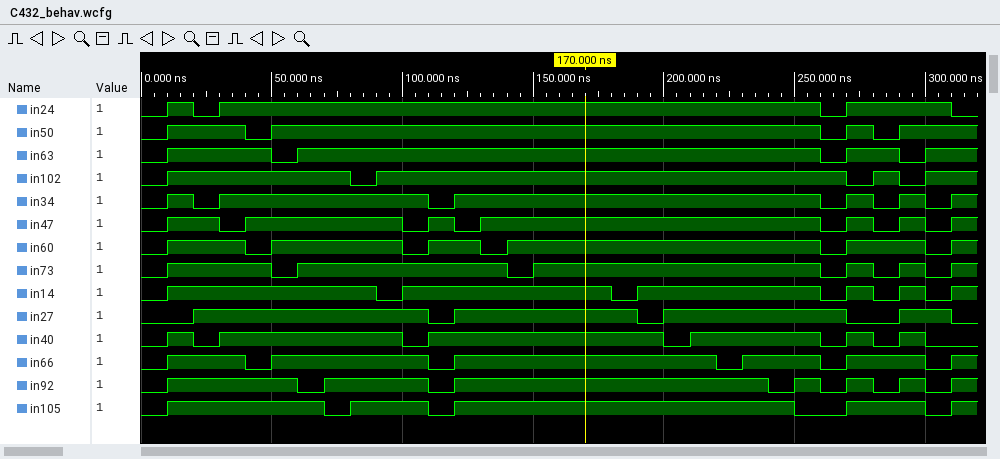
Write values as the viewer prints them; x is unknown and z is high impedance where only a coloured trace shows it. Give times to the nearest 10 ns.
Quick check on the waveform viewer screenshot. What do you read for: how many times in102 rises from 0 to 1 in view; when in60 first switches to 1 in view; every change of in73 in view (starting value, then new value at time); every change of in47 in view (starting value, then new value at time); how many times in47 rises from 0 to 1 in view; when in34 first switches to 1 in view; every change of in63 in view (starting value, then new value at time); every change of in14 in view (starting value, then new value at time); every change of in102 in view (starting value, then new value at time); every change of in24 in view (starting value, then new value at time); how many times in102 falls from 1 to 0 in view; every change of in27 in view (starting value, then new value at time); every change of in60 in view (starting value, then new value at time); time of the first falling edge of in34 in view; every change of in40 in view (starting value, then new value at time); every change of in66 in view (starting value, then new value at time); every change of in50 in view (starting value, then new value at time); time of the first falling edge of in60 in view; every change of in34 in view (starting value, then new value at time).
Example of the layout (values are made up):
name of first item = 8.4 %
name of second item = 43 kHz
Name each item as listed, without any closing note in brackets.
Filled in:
how many times in102 rises from 0 to 1 in view = 4
when in60 first switches to 1 in view = 10 ns
every change of in73 in view = 0, 1 at 10 ns, 0 at 50 ns, 1 at 60 ns, 0 at 140 ns, 1 at 150 ns, 0 at 260 ns, 1 at 270 ns, 0 at 280 ns, 1 at 290 ns, 0 at 300 ns, 1 at 310 ns
every change of in47 in view = 0, 1 at 10 ns, 0 at 30 ns, 1 at 40 ns, 0 at 100 ns, 1 at 110 ns, 0 at 120 ns, 1 at 130 ns, 0 at 260 ns, 1 at 270 ns, 0 at 280 ns, 1 at 290 ns, 0 at 300 ns, 1 at 310 ns
how many times in47 rises from 0 to 1 in view = 7
when in34 first switches to 1 in view = 10 ns
every change of in63 in view = 0, 1 at 10 ns, 0 at 50 ns, 1 at 60 ns, 0 at 260 ns, 1 at 270 ns, 0 at 290 ns, 1 at 300 ns
every change of in14 in view = 0, 1 at 10 ns, 0 at 90 ns, 1 at 100 ns, 0 at 180 ns, 1 at 190 ns, 0 at 260 ns, 1 at 270 ns, 0 at 280 ns, 1 at 290 ns, 0 at 300 ns, 1 at 310 ns
every change of in102 in view = 0, 1 at 10 ns, 0 at 80 ns, 1 at 90 ns, 0 at 270 ns, 1 at 280 ns, 0 at 290 ns, 1 at 300 ns
every change of in24 in view = 0, 1 at 10 ns, 0 at 20 ns, 1 at 30 ns, 0 at 260 ns, 1 at 270 ns, 0 at 310 ns
how many times in102 falls from 1 to 0 in view = 3
every change of in27 in view = 0, 1 at 20 ns, 0 at 110 ns, 1 at 120 ns, 0 at 190 ns, 1 at 200 ns, 0 at 270 ns, 1 at 290 ns, 0 at 310 ns
every change of in60 in view = 0, 1 at 10 ns, 0 at 40 ns, 1 at 50 ns, 0 at 100 ns, 1 at 110 ns, 0 at 130 ns, 1 at 140 ns, 0 at 260 ns, 1 at 270 ns, 0 at 300 ns, 1 at 310 ns
time of the first falling edge of in34 in view = 20 ns
every change of in40 in view = 0, 1 at 10 ns, 0 at 20 ns, 1 at 30 ns, 0 at 100 ns, 1 at 110 ns, 0 at 200 ns, 1 at 210 ns, 0 at 260 ns, 1 at 270 ns, 0 at 280 ns, 1 at 290 ns, 0 at 300 ns
every change of in66 in view = 0, 1 at 10 ns, 0 at 40 ns, 1 at 50 ns, 0 at 110 ns, 1 at 120 ns, 0 at 220 ns, 1 at 230 ns, 0 at 260 ns, 1 at 270 ns, 0 at 300 ns, 1 at 310 ns
every change of in50 in view = 0, 1 at 10 ns, 0 at 40 ns, 1 at 50 ns, 0 at 260 ns, 1 at 270 ns, 0 at 280 ns, 1 at 290 ns
time of the first falling edge of in60 in view = 40 ns
every change of in34 in view = 0, 1 at 10 ns, 0 at 20 ns, 1 at 30 ns, 0 at 110 ns, 1 at 120 ns, 0 at 260 ns, 1 at 270 ns, 0 at 280 ns, 1 at 290 ns, 0 at 300 ns, 1 at 310 ns
